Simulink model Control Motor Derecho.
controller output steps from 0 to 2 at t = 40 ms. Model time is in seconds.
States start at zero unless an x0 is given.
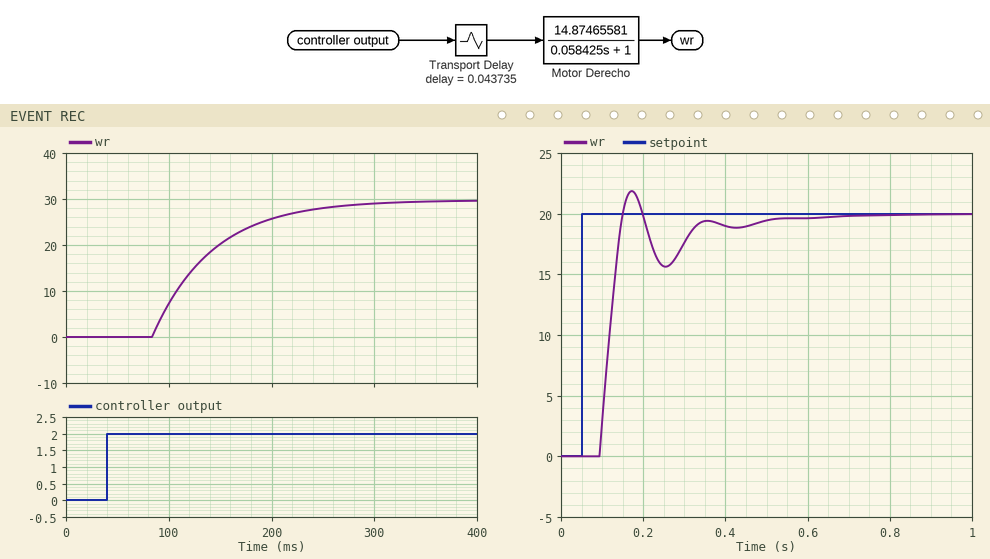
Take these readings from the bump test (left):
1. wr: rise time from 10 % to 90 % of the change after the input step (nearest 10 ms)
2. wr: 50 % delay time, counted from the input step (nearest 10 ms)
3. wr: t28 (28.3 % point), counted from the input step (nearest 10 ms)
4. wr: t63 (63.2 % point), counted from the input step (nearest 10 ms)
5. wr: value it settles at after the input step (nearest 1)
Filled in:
130 ms
80 ms
60 ms
100 ms
30
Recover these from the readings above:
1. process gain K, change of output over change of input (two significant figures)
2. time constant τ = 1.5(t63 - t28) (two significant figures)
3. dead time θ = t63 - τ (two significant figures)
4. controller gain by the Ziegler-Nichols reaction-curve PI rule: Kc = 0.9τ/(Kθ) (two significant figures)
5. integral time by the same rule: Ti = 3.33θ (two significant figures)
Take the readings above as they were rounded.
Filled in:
15
60 ms
40 ms
0.090
130 ms
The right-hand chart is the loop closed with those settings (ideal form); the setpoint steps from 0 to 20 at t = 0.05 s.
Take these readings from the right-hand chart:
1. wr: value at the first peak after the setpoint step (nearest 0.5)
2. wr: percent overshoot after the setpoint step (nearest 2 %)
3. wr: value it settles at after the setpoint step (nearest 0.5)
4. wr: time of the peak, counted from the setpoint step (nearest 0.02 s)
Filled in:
22.0
10 %
20.0
0.12 s
